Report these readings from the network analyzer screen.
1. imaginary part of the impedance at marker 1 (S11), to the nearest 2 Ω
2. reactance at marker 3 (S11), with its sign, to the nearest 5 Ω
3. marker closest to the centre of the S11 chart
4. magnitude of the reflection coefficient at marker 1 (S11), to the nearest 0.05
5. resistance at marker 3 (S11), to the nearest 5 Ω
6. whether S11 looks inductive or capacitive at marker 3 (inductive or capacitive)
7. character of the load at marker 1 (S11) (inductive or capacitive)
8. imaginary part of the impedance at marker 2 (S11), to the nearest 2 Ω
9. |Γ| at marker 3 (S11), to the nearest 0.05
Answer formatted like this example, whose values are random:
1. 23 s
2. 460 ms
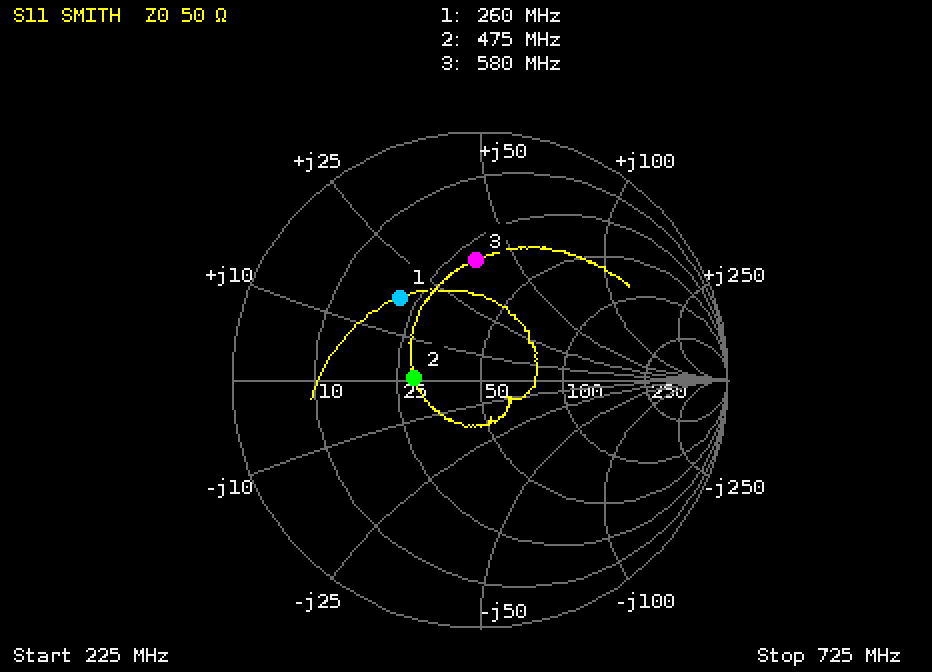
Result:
1. +18 Ω
2. +40 Ω
3. marker 2
4. 0.45
5. 30 Ω
6. inductive
7. inductive
8. 0 Ω
9. 0.50
